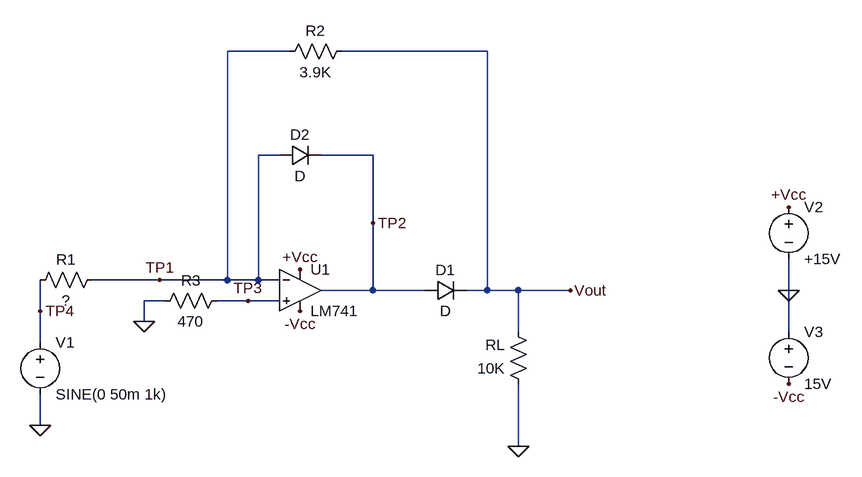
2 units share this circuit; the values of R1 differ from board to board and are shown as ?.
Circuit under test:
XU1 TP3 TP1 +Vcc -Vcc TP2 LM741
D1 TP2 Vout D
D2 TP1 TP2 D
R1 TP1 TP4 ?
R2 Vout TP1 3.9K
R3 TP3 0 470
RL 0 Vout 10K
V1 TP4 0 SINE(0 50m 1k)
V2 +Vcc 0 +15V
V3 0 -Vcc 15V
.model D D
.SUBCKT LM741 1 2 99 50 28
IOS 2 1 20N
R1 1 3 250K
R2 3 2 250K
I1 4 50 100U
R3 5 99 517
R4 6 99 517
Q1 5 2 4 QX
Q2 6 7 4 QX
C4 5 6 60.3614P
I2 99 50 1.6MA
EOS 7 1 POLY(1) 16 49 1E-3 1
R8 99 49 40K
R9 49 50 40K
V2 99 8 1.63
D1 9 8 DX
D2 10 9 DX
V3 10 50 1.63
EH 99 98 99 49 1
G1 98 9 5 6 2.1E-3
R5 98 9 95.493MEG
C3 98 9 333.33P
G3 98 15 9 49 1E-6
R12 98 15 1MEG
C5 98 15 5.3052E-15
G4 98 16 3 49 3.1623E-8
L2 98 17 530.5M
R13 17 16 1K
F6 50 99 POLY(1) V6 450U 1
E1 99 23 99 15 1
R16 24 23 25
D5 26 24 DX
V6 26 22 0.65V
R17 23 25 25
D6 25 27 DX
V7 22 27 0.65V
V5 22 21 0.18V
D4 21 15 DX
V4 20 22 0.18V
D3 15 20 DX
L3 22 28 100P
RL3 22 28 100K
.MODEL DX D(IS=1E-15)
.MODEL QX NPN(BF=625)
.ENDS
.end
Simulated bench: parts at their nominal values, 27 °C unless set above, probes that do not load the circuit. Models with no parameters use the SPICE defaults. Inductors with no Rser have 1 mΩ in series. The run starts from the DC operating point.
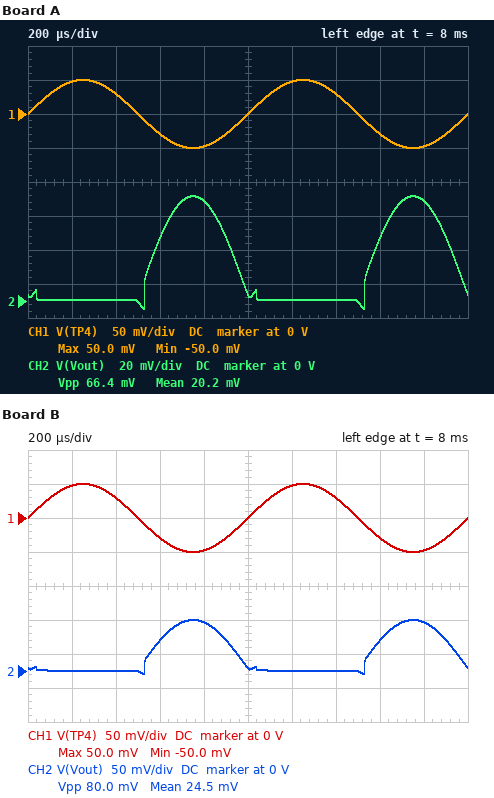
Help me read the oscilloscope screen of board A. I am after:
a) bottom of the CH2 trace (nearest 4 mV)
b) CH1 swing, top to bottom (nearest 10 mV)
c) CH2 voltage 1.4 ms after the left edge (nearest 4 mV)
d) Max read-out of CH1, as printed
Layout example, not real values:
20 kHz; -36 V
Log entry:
-4 mV; 100 mV; 0 V; 50.0 mV
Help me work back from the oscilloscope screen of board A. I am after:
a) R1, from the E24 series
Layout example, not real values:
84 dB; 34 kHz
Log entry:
3.3 kΩ
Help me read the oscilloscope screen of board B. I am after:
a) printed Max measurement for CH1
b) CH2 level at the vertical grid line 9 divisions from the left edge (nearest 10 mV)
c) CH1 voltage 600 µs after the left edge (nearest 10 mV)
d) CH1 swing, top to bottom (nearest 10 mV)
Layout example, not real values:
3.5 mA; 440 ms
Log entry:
50.0 mV; 70 mV; -30 mV; 100 mV
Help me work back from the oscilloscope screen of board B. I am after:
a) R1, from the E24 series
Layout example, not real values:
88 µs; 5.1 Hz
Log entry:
2.7 kΩ
